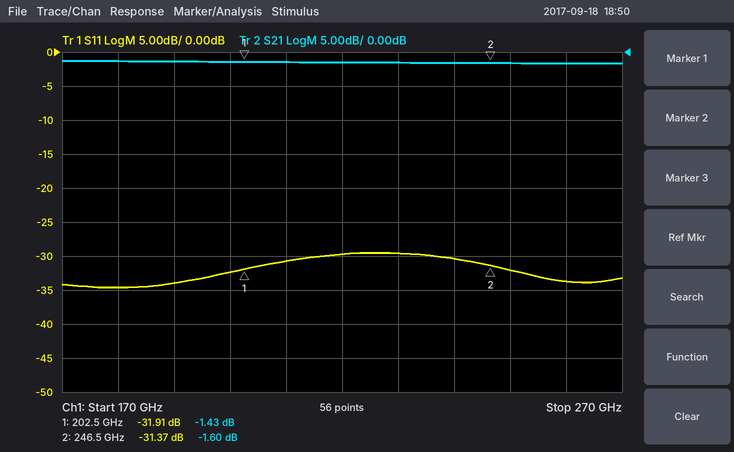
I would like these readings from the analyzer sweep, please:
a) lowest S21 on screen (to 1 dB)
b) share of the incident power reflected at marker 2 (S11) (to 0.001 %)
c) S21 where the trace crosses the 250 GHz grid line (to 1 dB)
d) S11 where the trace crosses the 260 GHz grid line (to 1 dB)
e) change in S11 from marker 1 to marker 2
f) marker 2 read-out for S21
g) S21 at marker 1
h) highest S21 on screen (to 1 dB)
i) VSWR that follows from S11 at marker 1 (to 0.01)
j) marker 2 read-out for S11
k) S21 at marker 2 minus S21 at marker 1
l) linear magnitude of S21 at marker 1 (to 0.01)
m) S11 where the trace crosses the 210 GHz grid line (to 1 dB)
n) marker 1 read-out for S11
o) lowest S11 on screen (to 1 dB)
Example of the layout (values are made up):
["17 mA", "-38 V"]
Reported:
["-2 dB", "0.073 %", "-2 dB", "-34 dB", "0.54 dB", "-1.60 dB", "-1.43 dB", "-1 dB", "1.05", "-31.37 dB", "-0.17 dB", "0.85", "-31 dB", "-31.91 dB", "-35 dB"]
